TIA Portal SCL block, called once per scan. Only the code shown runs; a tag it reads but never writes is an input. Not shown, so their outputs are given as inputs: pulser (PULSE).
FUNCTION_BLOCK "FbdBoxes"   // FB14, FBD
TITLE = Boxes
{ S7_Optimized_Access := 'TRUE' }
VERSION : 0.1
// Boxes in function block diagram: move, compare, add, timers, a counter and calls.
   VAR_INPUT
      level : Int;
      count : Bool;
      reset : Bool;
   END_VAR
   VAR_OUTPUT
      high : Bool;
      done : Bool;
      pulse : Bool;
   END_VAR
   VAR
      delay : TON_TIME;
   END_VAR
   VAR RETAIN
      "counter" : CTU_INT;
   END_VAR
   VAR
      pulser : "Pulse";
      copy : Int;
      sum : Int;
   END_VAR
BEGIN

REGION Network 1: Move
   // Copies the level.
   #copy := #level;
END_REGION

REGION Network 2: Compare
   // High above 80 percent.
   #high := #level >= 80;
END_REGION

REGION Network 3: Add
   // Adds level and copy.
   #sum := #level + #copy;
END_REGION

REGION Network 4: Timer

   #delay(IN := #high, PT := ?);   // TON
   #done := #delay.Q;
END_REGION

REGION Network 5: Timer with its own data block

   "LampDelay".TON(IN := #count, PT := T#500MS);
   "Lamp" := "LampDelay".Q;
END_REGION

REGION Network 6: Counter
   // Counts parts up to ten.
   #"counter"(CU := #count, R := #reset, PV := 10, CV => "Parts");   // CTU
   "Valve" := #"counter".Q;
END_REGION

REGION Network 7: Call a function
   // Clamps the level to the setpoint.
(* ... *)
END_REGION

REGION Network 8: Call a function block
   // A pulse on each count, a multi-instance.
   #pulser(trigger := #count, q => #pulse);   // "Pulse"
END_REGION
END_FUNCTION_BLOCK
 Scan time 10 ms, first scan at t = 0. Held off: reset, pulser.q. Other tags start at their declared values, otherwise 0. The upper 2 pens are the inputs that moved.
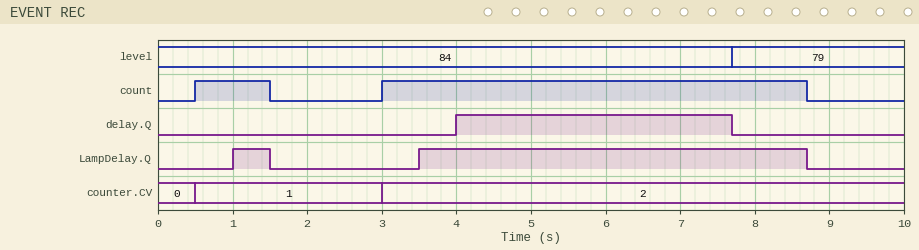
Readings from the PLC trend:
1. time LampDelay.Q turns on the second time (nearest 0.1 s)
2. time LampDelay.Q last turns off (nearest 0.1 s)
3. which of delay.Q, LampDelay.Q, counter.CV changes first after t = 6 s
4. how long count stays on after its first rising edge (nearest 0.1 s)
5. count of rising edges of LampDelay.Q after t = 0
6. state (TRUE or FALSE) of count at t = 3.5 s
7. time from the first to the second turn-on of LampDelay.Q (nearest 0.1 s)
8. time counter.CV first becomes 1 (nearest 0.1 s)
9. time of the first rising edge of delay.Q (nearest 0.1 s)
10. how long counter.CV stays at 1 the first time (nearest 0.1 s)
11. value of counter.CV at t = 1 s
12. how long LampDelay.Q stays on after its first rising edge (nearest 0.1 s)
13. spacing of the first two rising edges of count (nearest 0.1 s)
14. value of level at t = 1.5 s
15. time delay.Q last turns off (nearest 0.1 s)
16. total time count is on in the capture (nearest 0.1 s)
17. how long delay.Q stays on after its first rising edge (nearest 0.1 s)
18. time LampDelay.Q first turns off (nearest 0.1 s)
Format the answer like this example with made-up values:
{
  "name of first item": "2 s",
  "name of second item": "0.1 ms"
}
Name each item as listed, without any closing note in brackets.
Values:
{
  "time LampDelay.Q turns on the second time": "3.5 s",
  "time LampDelay.Q last turns off": "8.7 s",
  "which of delay.Q, LampDelay.Q, counter.CV changes first after t = 6 s": "delay.Q",
  "how long count stays on after its first rising edge": "1.0 s",
  "count of rising edges of LampDelay.Q after t = 0": "2",
  "state (TRUE or FALSE) of count at t = 3.5 s": "TRUE",
  "time from the first to the second turn-on of LampDelay.Q": "2.5 s",
  "time counter.CV first becomes 1": "0.5 s",
  "time of the first rising edge of delay.Q": "4.0 s",
  "how long counter.CV stays at 1 the first time": "2.5 s",
  "value of counter.CV at t = 1 s": "1",
  "how long LampDelay.Q stays on after its first rising edge": "0.5 s",
  "spacing of the first two rising edges of count": "2.5 s",
  "value of level at t = 1.5 s": "84",
  "time delay.Q last turns off": "7.7 s",
  "total time count is on in the capture": "6.7 s",
  "how long delay.Q stays on after its first rising edge": "3.7 s",
  "time LampDelay.Q first turns off": "1.5 s"
}
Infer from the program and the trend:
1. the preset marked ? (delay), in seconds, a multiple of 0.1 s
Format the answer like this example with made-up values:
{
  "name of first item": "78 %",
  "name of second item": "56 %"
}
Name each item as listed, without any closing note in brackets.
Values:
{
  "the preset marked ? (delay), in seconds, a multiple of 0.1 s": "4.0 s"
}
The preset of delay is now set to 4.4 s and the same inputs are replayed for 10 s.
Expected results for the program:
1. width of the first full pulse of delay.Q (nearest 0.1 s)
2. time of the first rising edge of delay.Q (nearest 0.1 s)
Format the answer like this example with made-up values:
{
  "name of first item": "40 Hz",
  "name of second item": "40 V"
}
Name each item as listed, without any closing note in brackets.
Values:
{
  "width of the first full pulse of delay.Q": "3.3 s",
  "time of the first rising edge of delay.Q": "4.4 s"
}
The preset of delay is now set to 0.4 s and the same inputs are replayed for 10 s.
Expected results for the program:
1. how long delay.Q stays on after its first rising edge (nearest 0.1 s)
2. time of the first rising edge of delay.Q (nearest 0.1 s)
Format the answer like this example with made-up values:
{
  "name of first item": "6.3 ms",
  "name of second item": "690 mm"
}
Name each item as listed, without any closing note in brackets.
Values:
{
  "how long delay.Q stays on after its first rising edge": "7.3 s",
  "time of the first rising edge of delay.Q": "0.4 s"
}
